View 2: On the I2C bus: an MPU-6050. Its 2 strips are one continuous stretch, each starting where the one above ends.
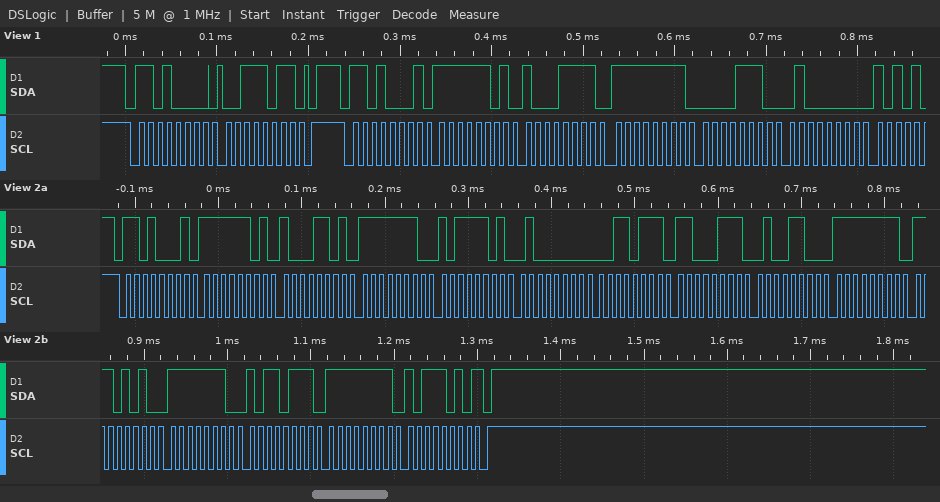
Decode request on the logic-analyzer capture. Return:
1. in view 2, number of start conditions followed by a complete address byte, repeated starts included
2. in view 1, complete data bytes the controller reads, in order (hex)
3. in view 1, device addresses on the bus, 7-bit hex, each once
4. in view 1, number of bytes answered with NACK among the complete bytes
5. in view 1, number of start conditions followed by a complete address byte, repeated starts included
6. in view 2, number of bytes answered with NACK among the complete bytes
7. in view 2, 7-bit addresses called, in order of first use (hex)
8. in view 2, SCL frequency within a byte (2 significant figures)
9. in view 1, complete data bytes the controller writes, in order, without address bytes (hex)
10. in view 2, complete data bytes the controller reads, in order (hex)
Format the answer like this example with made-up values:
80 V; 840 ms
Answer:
1; FD 8F FF 0E 40; 0x68; 0; 2; 1; 0x68; 100 kHz; 3B; FD 8D FE BD 40 37 C7 4C FF EA FE B7 FF BA
